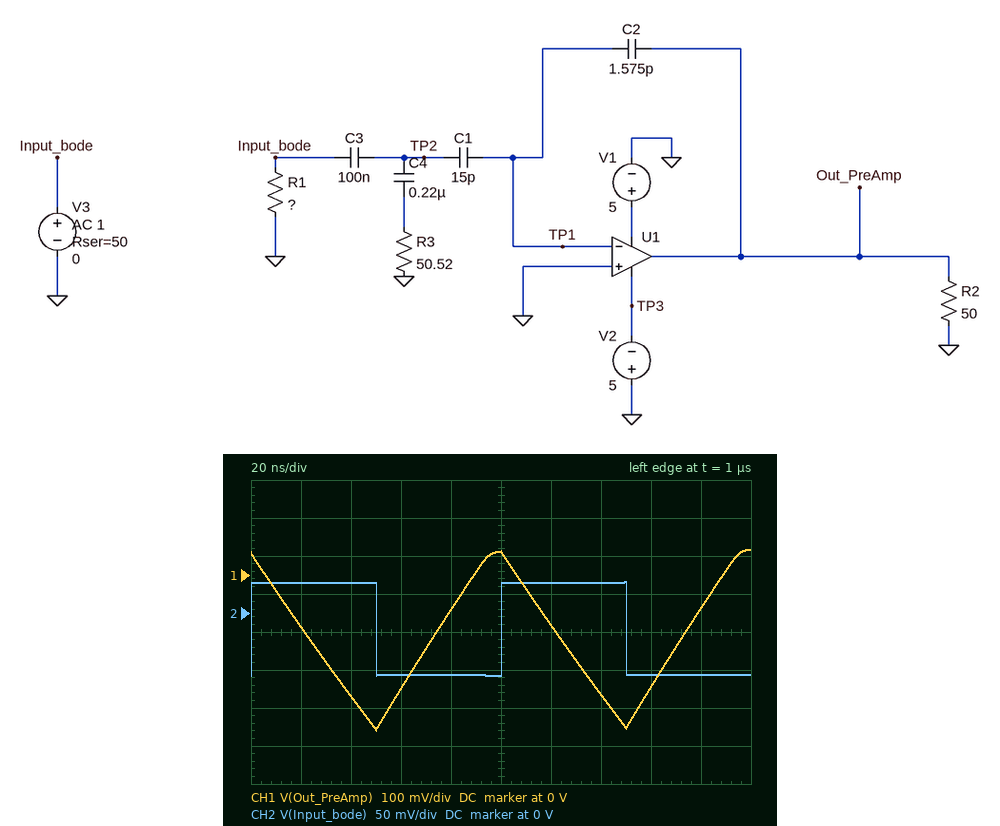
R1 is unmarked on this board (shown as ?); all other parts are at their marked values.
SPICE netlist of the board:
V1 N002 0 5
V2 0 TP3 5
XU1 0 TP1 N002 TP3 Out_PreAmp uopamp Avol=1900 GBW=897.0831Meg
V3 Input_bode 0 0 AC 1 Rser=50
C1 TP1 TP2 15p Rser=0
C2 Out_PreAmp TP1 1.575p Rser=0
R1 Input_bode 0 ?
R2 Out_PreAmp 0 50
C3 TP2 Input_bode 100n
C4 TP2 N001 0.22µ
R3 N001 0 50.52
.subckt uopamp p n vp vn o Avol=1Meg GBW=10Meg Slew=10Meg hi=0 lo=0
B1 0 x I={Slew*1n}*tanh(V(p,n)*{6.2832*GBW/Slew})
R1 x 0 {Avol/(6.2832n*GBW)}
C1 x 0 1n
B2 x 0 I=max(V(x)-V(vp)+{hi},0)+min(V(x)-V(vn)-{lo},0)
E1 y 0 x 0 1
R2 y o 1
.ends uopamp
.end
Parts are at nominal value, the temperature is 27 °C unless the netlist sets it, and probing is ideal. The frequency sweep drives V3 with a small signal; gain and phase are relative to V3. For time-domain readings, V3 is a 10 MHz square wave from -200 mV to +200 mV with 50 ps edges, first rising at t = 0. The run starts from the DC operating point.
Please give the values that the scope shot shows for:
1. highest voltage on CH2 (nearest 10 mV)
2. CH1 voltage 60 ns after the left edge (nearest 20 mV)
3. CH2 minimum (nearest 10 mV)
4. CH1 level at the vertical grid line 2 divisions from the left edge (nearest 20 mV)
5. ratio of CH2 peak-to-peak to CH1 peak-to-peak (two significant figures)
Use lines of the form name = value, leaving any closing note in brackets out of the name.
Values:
highest voltage on CH2 = 40 mV
CH1 voltage 60 ns after the left edge = -300 mV
CH2 minimum = -80 mV
CH1 level at the vertical grid line 2 divisions from the left edge = -320 mV
ratio of CH2 peak-to-peak to CH1 peak-to-peak = 0.26
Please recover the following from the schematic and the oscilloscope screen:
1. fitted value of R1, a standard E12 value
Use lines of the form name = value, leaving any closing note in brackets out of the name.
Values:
fitted value of R1, a standard E12 value = 39 Ω
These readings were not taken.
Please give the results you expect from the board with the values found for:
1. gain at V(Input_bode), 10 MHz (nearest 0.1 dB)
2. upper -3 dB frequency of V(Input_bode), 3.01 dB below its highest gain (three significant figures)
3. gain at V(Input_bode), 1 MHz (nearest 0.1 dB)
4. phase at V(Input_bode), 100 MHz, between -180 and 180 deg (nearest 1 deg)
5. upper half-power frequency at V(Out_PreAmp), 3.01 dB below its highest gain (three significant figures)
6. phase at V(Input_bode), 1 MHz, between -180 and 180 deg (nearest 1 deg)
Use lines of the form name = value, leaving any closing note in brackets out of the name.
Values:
gain at V(Input_bode), 10 MHz = -10.3 dB
upper -3 dB frequency of V(Input_bode), 3.01 dB below its highest gain = 195 kHz
gain at V(Input_bode), 1 MHz = -10.3 dB
phase at V(Input_bode), 100 MHz, between -180 and 180 deg = -4 deg
upper half-power frequency at V(Out_PreAmp), 3.01 dB below its highest gain = 75.8 MHz
phase at V(Input_bode), 1 MHz, between -180 and 180 deg = -1 deg
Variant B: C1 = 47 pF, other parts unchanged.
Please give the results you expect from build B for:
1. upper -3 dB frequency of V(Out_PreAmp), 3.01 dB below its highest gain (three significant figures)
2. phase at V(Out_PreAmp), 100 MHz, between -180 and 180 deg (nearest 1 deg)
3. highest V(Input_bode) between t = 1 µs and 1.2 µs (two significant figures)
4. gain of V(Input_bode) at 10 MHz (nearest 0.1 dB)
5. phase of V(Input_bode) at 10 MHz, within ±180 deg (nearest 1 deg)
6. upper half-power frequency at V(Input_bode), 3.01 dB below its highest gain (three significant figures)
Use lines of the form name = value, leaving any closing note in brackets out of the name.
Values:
upper -3 dB frequency of V(Out_PreAmp), 3.01 dB below its highest gain = 25.8 MHz
phase at V(Out_PreAmp), 100 MHz, between -180 and 180 deg = 104 deg
highest V(Input_bode) between t = 1 µs and 1.2 µs = 40 mV
gain of V(Input_bode) at 10 MHz = -10.4 dB
phase of V(Input_bode) at 10 MHz, within ±180 deg = -2 deg
upper half-power frequency at V(Input_bode), 3.01 dB below its highest gain = 196 kHz
